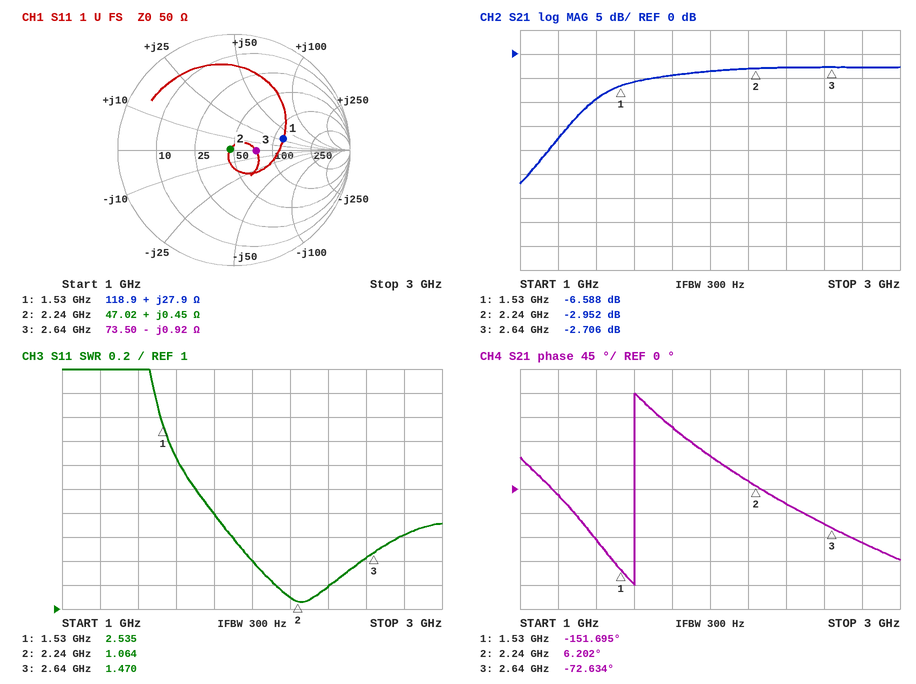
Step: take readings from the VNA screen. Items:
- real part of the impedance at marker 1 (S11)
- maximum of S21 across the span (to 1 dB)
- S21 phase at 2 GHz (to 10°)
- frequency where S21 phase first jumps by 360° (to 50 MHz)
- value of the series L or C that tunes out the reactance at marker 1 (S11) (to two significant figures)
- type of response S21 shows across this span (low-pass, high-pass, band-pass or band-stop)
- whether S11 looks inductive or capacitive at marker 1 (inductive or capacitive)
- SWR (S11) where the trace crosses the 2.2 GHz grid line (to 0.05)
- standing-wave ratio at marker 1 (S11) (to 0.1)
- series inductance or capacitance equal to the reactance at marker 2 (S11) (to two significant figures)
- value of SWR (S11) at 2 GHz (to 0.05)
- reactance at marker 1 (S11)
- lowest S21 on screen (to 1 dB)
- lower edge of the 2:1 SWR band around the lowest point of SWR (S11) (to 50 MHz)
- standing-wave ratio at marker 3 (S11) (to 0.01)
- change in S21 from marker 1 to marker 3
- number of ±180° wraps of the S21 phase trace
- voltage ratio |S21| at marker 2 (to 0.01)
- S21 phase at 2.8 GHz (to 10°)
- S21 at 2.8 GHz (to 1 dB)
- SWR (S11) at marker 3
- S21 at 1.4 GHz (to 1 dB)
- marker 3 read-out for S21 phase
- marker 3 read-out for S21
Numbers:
118.9 Ω
-3 dB
60°
1.60 GHz
3.7 pF
high-pass
inductive
1.10
2.5
32 pH
1.40
+27.9 Ω
-27 dB
1.70 GHz
1.47
3.882 dB
1
0.71
-100°
-3 dB
1.470
-9 dB
-72.634°
-2.706 dB
